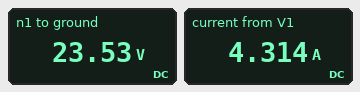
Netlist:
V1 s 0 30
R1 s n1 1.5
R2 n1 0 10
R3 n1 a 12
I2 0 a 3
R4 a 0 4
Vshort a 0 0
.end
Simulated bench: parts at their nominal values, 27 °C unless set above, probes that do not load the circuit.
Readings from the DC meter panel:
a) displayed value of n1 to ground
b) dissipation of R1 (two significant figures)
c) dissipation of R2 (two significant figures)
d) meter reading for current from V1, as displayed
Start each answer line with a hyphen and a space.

- 23.53 V
- 28 W
- 55 W
- 4.314 A
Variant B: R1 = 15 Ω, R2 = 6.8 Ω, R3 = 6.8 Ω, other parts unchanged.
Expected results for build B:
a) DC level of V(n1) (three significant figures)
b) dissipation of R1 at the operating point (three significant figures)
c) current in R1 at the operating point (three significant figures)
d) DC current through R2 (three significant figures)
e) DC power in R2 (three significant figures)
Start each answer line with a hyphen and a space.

- 5.54 V
- 39.9 W
- 1.63 A
- 815 mA
- 4.52 W
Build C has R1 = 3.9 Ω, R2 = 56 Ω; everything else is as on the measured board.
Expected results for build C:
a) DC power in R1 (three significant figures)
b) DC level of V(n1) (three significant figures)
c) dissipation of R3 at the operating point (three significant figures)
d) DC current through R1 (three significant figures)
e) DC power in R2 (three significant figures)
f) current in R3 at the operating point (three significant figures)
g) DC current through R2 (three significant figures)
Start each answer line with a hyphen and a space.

- 18.5 W
- 21.5 V
- 38.6 W
- 2.18 A
- 8.26 W
- 1.79 A
- 384 mA
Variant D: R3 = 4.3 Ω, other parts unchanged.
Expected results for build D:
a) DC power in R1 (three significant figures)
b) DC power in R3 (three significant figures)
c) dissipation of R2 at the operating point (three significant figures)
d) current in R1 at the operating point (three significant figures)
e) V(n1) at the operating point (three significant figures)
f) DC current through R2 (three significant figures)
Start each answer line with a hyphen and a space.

- 66.5 W
- 93.2 W
- 40.1 W
- 6.66 A
- 20.0 V
- 2.00 A
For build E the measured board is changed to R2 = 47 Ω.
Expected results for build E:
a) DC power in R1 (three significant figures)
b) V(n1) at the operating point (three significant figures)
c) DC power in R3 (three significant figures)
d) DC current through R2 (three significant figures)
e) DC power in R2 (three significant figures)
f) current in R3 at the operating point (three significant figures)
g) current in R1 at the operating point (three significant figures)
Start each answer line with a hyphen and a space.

- 11.0 W
- 25.9 V
- 56.0 W
- 552 mA
- 14.3 W
- 2.16 A
- 2.71 A
